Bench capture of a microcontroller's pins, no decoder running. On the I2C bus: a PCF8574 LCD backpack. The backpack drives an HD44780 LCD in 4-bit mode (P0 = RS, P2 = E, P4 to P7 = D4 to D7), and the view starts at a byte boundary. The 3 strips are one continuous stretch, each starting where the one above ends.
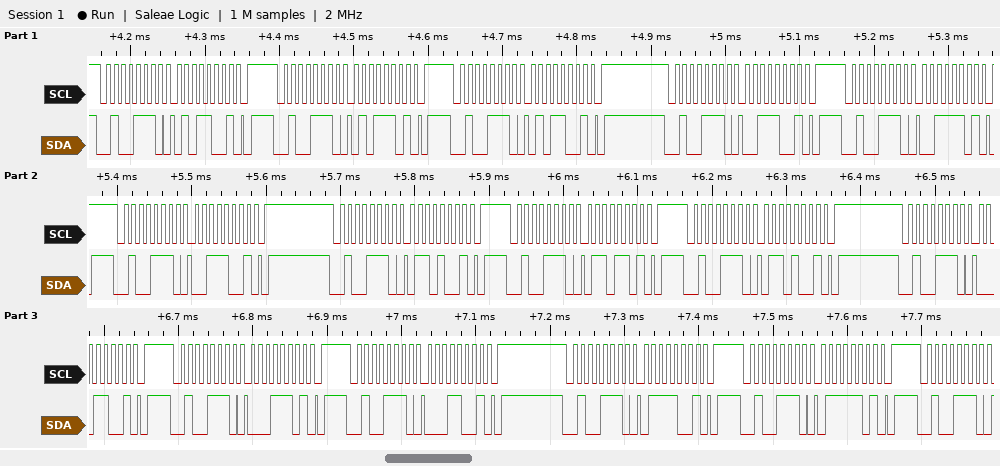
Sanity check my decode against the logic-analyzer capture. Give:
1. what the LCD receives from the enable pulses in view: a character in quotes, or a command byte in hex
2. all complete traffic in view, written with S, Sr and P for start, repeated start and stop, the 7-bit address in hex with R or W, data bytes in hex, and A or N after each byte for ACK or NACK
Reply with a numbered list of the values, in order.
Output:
1. 'S' 'a'
2. S 27W A 59 A P S 27W A 5D A P S 27W A 59 A P S 27W A 39 A P S 27W A 3D A P S 27W A 39 A P S 27W A 69 A P S 27W A 6D A P S 27W A 69 A P S 27W A 19 A P S 27W A 1D A P S 27W A 19 A P S 27W A 79 A P S 27W A 7D A P S 27W A
